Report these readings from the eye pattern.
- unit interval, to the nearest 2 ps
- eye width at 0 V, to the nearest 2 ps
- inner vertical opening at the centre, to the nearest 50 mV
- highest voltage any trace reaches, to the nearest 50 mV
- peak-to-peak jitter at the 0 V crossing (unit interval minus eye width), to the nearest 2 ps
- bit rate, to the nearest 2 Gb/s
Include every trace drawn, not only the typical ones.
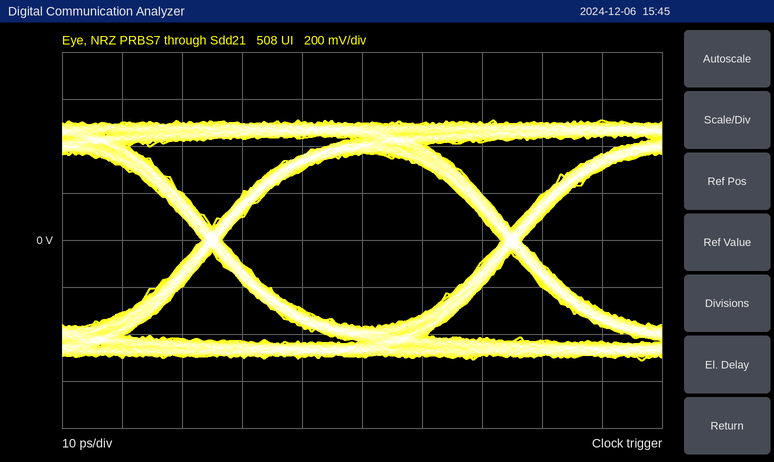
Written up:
50 ps
46 ps
750 mV
500 mV
4 ps
20 Gb/s
